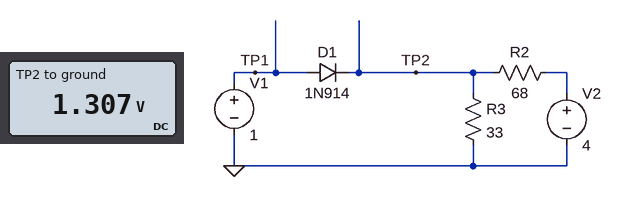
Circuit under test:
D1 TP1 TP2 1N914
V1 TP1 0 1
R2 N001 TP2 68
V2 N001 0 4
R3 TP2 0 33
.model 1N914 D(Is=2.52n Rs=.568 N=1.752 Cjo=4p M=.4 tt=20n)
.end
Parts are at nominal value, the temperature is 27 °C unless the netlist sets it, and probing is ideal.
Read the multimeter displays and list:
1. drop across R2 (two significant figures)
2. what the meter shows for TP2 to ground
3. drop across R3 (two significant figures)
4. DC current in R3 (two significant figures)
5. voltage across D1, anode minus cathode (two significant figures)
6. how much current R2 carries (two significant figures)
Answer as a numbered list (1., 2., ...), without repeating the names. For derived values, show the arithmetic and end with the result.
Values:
1. 4 V - 1.307 V = 2.7 V
2. 1.307 V
3. 1.307 V = 1.3 V
4. (1.307 V) / 33 Ω = 40 mA
5. 1 V - 1.307 V = -310 mV
6. (4 V - 1.307 V) / 68 Ω = 40 mA
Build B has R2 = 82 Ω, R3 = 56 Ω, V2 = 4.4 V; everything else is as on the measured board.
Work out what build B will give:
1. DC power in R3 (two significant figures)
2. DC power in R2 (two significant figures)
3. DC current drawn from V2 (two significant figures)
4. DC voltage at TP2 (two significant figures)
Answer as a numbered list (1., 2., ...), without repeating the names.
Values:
1. 57 mW
2. 83 mW
3. 32 mA
4. 1.8 V
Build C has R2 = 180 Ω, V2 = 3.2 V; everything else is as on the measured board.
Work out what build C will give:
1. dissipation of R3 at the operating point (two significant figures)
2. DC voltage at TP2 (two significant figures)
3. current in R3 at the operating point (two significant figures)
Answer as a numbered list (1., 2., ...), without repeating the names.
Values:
1. 7.6 mW
2. 500 mV
3. 15 mA
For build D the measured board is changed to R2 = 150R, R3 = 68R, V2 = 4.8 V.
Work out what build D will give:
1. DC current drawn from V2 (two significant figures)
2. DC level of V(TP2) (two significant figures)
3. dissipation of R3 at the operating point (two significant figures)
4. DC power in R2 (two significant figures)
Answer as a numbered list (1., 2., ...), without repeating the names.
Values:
1. 22 mA
2. 1.5 V
3. 33 mW
4. 73 mW
